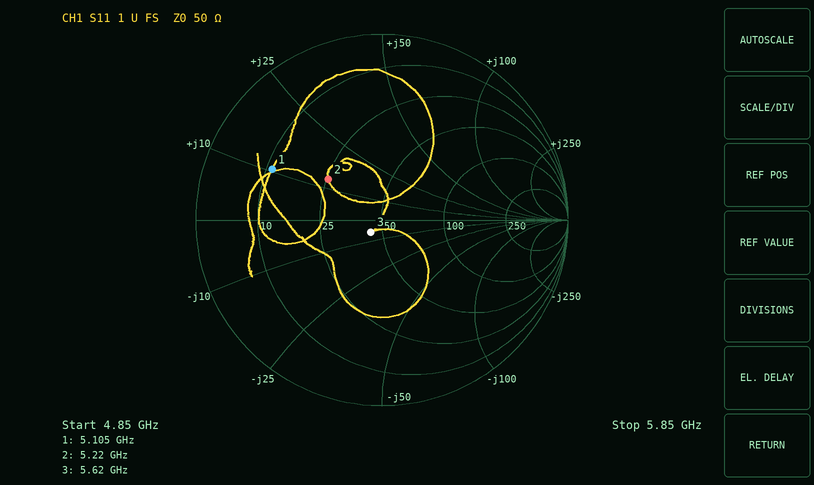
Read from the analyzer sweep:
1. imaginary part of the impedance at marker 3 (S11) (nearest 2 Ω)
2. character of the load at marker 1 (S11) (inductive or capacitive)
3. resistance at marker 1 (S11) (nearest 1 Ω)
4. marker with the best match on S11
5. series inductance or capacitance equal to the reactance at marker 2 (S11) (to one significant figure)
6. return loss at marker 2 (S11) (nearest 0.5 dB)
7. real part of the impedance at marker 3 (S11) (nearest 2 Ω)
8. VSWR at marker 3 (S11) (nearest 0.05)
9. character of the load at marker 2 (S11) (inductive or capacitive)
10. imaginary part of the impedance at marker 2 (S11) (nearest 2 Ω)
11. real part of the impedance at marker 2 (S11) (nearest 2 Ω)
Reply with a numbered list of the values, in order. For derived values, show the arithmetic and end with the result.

1. -6 Ω
2. inductive
3. 11 Ω
4. marker 3
5. L = 12 Ω/(2π × 5.22 GHz) ≈ 366 pH, so 400 pH to one significant figure
6. 9.0 dB
7. 44 Ω
8. 1.20
9. inductive
10. +12 Ω
11. 26 Ω
